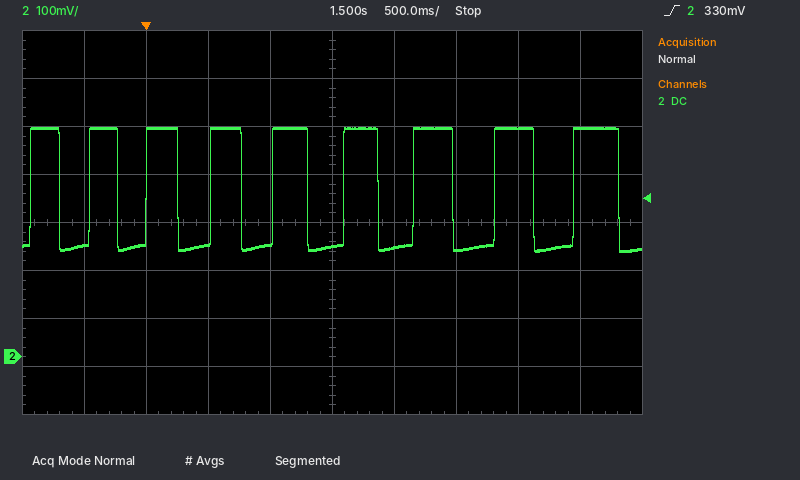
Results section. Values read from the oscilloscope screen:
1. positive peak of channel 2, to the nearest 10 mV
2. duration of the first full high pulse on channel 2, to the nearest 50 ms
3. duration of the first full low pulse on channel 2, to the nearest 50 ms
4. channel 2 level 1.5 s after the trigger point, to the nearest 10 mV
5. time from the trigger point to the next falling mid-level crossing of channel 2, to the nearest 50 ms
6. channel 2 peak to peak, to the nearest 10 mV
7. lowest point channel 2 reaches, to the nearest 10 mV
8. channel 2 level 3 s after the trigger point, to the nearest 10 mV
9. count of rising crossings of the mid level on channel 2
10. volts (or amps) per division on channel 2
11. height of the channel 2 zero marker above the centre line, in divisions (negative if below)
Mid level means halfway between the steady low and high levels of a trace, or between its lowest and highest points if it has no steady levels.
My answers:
480 mV
250 ms
250 ms
230 mV
250 ms
260 mV
220 mV
480 mV
9
100 mV
-2.8 div
